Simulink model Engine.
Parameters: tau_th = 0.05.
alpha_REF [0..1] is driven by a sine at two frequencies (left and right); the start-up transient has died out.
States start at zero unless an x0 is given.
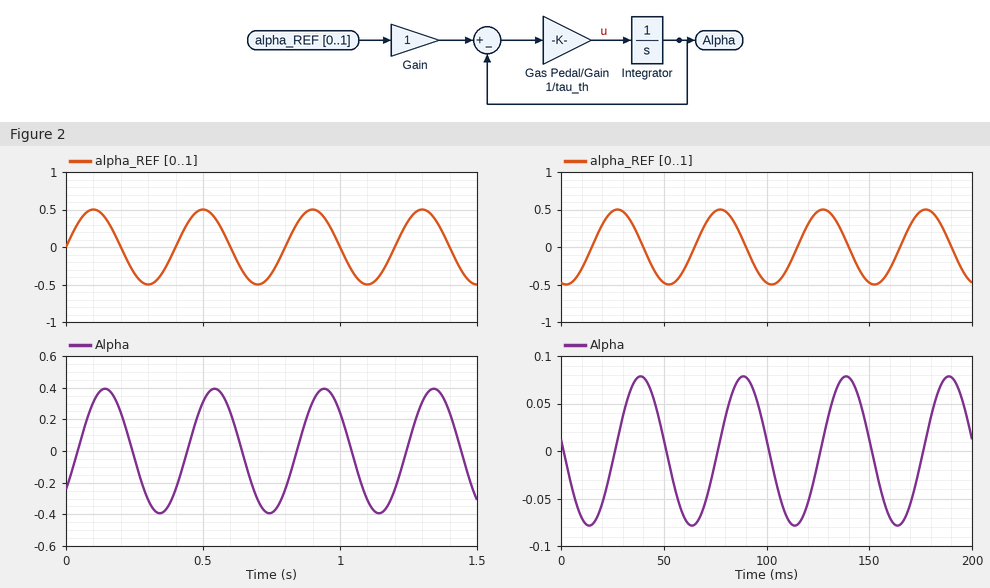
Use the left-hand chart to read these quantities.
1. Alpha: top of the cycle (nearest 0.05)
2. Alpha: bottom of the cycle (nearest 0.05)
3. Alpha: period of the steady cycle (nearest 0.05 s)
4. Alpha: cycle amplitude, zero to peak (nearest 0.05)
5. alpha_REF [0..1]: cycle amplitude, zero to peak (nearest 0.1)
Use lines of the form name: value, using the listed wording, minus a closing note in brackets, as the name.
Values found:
Alpha: top of the cycle: 0.40
Alpha: bottom of the cycle: -0.40
Alpha: period of the steady cycle: 0.40 s
Alpha: cycle amplitude, zero to peak: 0.40
alpha_REF [0..1]: cycle amplitude, zero to peak: 0.5
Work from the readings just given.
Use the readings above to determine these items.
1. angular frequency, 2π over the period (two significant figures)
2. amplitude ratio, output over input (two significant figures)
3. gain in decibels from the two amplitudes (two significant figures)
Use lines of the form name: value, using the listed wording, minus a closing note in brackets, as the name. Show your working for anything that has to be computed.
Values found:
angular frequency, 2π over the period: 2π / 0.4 = 16 rad/s
amplitude ratio, output over input: 0.4 / 0.5 = 0.80
gain in decibels from the two amplitudes: 20 log10(0.4 / 0.5) = -1.9 dB
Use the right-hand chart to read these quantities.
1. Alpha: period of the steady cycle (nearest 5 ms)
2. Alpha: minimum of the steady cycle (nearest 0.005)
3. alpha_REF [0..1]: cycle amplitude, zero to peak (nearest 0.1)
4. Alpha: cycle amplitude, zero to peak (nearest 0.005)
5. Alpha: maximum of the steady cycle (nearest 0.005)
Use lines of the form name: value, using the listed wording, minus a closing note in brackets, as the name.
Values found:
Alpha: period of the steady cycle: 50 ms
Alpha: minimum of the steady cycle: -0.080
alpha_REF [0..1]: cycle amplitude, zero to peak: 0.5
Alpha: cycle amplitude, zero to peak: 0.080
Alpha: maximum of the steady cycle: 0.080
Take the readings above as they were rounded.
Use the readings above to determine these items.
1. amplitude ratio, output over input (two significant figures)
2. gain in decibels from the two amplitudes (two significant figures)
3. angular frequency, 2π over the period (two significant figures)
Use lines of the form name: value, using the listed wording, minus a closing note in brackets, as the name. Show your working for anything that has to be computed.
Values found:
amplitude ratio, output over input: 0.08 / 0.5 = 0.16
gain in decibels from the two amplitudes: 20 log10(0.08 / 0.5) = -16 dB
angular frequency, 2π over the period: 2π / 50 = 0.13 rad/ms
